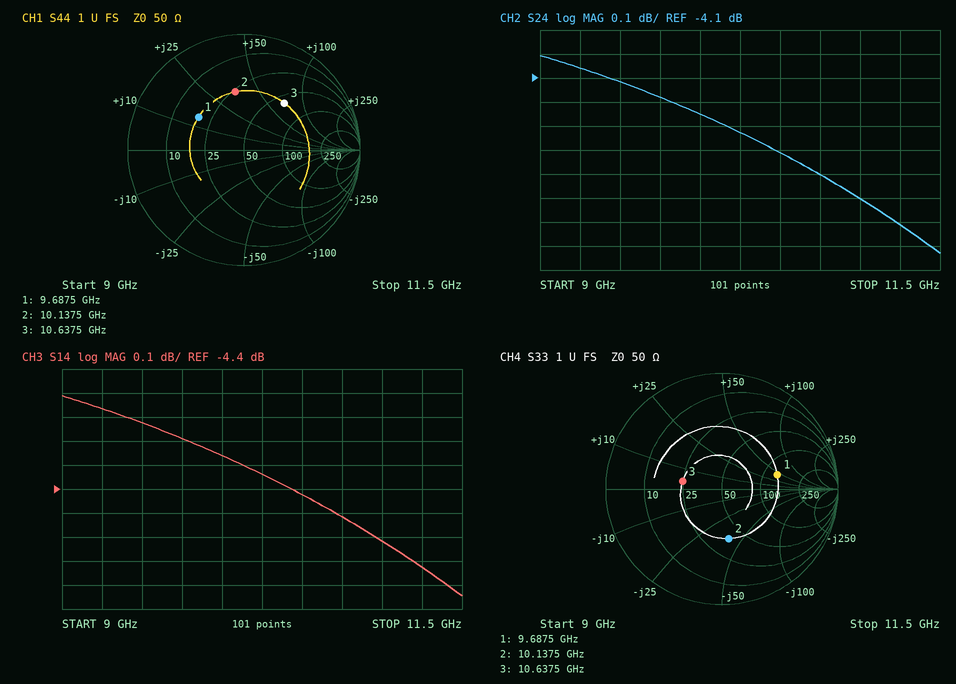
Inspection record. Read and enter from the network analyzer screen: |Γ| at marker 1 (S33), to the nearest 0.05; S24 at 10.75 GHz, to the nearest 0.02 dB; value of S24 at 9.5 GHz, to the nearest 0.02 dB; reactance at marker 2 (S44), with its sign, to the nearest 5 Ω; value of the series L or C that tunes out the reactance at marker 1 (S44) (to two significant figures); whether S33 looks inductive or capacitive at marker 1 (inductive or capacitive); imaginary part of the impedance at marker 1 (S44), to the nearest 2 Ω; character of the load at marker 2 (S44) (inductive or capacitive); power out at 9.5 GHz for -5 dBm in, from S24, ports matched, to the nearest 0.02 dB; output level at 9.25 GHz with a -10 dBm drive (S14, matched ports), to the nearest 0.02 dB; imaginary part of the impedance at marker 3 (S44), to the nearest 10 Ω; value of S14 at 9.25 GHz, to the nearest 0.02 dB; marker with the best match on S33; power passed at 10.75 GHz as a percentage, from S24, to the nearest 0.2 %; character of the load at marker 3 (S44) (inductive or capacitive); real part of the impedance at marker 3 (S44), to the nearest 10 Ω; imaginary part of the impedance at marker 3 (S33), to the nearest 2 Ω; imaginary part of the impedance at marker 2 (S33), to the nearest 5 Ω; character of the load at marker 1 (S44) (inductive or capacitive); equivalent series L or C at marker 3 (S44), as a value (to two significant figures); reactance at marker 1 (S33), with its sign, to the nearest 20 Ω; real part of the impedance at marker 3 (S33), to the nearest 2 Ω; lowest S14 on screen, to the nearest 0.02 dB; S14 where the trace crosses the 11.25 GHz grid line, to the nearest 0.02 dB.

0.50
-4.50 dB
-4.12 dB
+35 Ω
1.2 pF
inductive
+14 Ω
inductive
-9.12 dBm
-14.06 dBm
+70 Ω
-4.06 dB
marker 3
35.4 %
inductive
60 Ω
+4 Ω
-40 Ω
inductive
1.0 nH
+40 Ω
24 Ω
-4.84 dB
-4.72 dB
